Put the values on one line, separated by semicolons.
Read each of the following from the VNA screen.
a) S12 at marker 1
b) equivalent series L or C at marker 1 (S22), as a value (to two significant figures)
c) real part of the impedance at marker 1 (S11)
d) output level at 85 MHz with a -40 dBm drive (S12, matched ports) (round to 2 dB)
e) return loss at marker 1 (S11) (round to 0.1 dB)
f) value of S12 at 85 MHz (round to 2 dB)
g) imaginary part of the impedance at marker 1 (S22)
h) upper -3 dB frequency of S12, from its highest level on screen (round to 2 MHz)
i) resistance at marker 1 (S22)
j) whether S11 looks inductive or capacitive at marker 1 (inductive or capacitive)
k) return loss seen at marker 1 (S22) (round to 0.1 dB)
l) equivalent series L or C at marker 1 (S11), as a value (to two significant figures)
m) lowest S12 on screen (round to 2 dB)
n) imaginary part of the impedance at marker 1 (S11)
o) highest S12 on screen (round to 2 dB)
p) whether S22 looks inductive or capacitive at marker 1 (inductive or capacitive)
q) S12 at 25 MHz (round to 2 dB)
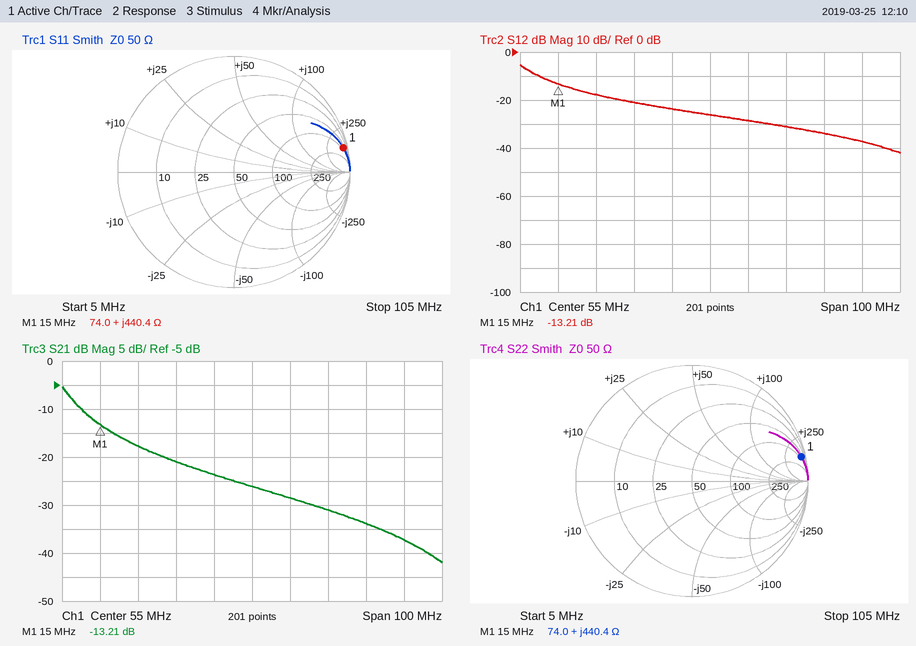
-13.21 dB; 4.7 µH; 74.0 Ω; -74 dBm; 0.3 dB; -34 dB; +440.4 Ω; 8 MHz; 74.0 Ω; inductive; 0.3 dB; 4.7 µH; -42 dB; +440.4 Ω; -6 dB; inductive; -18 dB
